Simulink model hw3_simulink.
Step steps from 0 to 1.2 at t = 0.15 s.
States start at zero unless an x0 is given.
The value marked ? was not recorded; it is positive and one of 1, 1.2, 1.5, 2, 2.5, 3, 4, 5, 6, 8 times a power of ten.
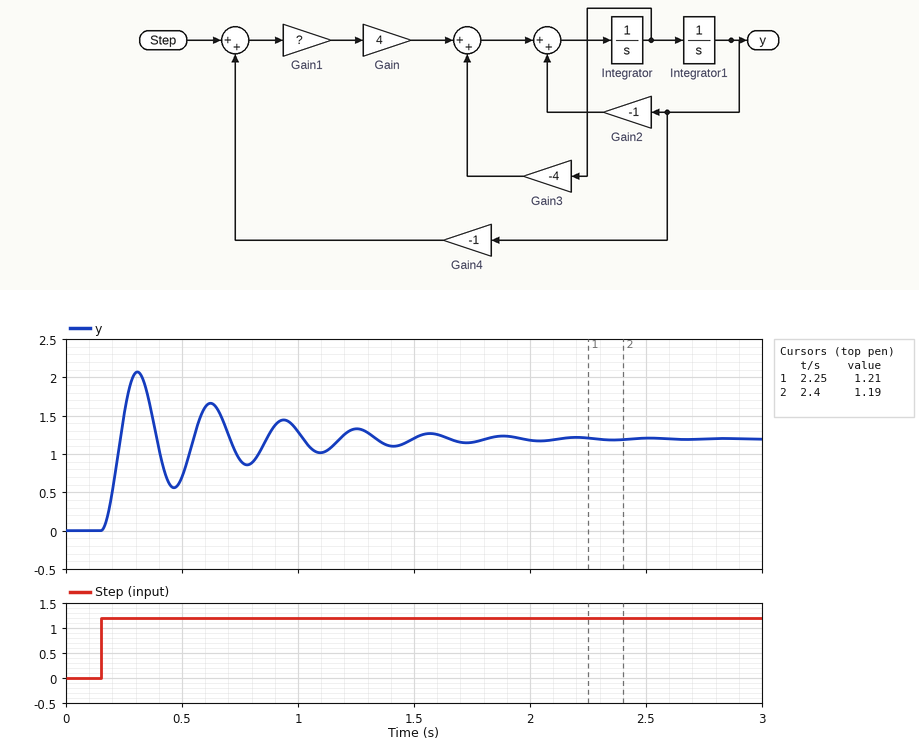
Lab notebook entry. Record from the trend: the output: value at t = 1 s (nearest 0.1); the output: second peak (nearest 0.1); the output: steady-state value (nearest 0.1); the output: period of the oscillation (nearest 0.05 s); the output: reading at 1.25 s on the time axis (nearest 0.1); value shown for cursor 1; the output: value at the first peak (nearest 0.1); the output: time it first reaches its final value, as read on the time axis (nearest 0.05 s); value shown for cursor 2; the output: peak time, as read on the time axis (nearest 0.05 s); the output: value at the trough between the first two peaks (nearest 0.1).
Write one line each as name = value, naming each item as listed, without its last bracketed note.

the output: value at t = 1 s = 1.3
the output: second peak = 1.7
the output: steady-state value = 1.2
the output: period of the oscillation = 0.30 s
the output: reading at 1.25 s on the time axis = 1.3
value shown for cursor 1 = 1.21
the output: value at the first peak = 2.1
the output: time it first reaches its final value, as read on the time axis = 0.25 s
value shown for cursor 2 = 1.19
the output: peak time, as read on the time axis = 0.30 s
the output: value at the trough between the first two peaks = 0.6
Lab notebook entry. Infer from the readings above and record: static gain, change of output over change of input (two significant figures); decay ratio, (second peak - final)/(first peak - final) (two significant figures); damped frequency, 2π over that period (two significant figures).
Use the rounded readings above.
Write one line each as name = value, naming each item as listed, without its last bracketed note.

static gain, change of output over change of input = 1.0
decay ratio, (second peak - final)/(first peak - final) = 0.56
damped frequency, 2π over that period = 21 rad/s
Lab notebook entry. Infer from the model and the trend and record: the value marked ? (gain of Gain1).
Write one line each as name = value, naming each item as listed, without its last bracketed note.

the value marked ? = 100
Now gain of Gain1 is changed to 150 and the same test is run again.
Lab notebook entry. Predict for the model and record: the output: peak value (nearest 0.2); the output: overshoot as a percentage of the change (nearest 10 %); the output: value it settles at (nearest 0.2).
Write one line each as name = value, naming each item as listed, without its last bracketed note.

the output: peak value = 2.2
the output: overshoot as a percentage of the change = 80 %
the output: value it settles at = 1.2
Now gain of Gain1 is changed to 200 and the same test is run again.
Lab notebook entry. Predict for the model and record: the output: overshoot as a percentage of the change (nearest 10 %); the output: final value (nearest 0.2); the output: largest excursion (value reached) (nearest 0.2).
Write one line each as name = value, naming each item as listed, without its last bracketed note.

the output: overshoot as a percentage of the change = 80 %
the output: final value = 1.2
the output: largest excursion (value reached) = 2.2
